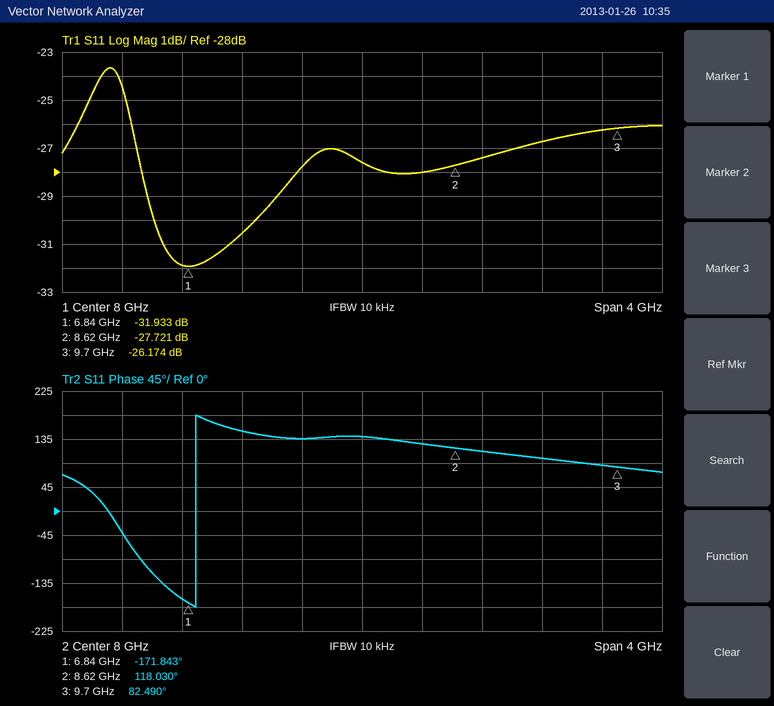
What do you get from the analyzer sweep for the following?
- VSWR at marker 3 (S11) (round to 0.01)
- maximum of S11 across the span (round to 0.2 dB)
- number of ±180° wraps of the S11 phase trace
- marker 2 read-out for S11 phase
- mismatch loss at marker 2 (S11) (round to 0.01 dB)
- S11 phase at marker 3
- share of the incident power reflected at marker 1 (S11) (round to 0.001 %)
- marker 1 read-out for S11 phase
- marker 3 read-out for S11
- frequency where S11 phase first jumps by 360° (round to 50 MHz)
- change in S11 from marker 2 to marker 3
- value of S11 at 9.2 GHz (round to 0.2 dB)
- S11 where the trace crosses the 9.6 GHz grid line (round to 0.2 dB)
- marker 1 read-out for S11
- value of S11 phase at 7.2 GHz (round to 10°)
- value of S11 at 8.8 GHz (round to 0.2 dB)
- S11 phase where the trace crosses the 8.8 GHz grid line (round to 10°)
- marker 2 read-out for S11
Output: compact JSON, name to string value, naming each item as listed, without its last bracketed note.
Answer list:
{"VSWR at marker 3 (S11)": "1.10", "maximum of S11 across the span": "-23.6 dB", "number of ±180° wraps of the S11 phase trace": "1", "marker 2 read-out for S11 phase": "118.030°", "mismatch loss at marker 2 (S11)": "0.01 dB", "S11 phase at marker 3": "82.490°", "share of the incident power reflected at marker 1 (S11)": "0.064 %", "marker 1 read-out for S11 phase": "-171.843°", "marker 3 read-out for S11": "-26.174 dB", "frequency where S11 phase first jumps by 360°": "6.90 GHz", "change in S11 from marker 2 to marker 3": "1.547 dB", "value of S11 at 9.2 GHz": "-26.8 dB", "S11 where the trace crosses the 9.6 GHz grid line": "-26.2 dB", "marker 1 read-out for S11": "-31.933 dB", "value of S11 phase at 7.2 GHz": "150°", "value of S11 at 8.8 GHz": "-27.4 dB", "S11 phase where the trace crosses the 8.8 GHz grid line": "110°", "marker 2 read-out for S11": "-27.721 dB"}
